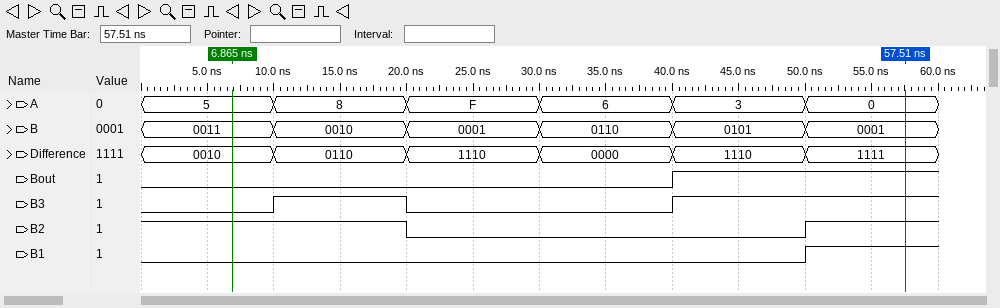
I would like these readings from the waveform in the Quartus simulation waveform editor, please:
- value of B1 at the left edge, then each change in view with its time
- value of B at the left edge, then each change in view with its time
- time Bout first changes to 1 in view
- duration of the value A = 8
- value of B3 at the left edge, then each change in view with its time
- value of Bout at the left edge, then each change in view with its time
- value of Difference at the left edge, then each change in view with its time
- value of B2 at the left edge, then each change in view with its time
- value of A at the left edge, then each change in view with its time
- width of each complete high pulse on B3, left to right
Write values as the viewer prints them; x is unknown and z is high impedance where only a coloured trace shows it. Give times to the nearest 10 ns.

0, 1 at 50 ns
0011, 0010 at 10 ns, 0001 at 20 ns, 0110 at 30 ns, 0101 at 40 ns, 0001 at 50 ns
40 ns
10 ns
0, 1 at 10 ns, 0 at 20 ns, 1 at 40 ns
0, 1 at 40 ns
0010, 0110 at 10 ns, 1110 at 20 ns, 0000 at 30 ns, 1110 at 40 ns, 1111 at 50 ns
1, 0 at 20 ns, 1 at 50 ns
5, 8 at 10 ns, F at 20 ns, 6 at 30 ns, 3 at 40 ns, 0 at 50 ns
10 ns
